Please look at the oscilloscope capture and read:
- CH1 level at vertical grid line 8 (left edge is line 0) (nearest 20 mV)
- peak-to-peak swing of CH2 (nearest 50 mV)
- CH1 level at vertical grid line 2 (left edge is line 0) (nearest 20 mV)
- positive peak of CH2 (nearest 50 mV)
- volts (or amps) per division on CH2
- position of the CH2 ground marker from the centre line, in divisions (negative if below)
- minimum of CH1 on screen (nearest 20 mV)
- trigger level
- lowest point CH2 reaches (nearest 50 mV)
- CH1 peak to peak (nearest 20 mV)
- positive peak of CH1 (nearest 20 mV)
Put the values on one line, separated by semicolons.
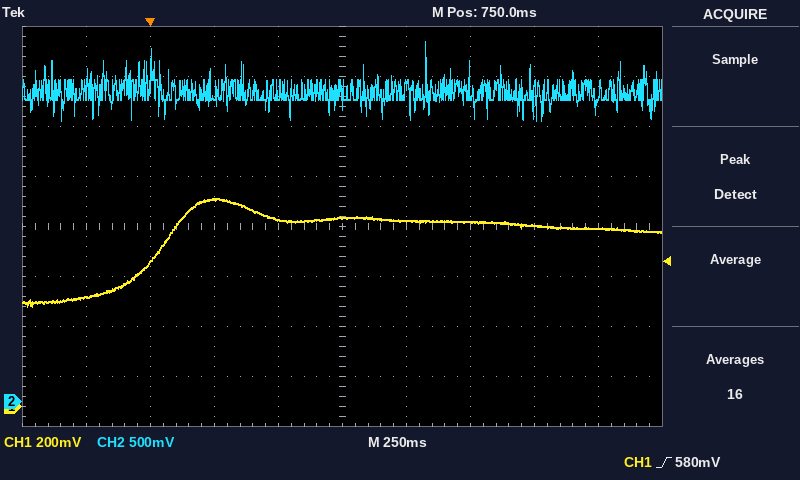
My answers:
720 mV; 800 mV; 580 mV; 3.60 V; 500 mV; -3.5 div; 400 mV; 580 mV; 2.80 V; 440 mV; 840 mV
